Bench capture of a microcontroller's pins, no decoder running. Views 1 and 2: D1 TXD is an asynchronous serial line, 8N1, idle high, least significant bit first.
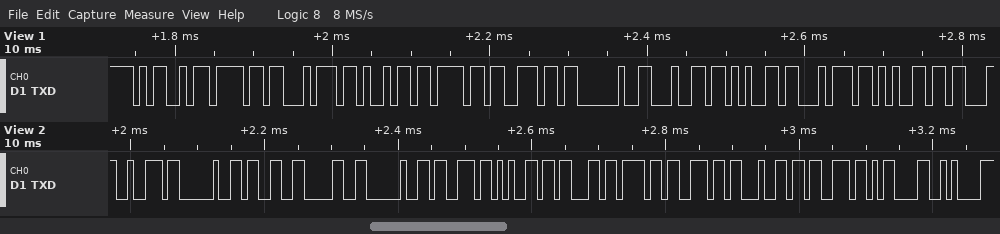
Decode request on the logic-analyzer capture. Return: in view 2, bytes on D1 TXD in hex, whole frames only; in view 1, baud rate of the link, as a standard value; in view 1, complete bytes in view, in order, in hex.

72 20 33 30 20 73 65 63 6F 6E 64 73 0D 0A
115200 baud
4D 6F 74 69 6F 6E 20 64 65 74 65
